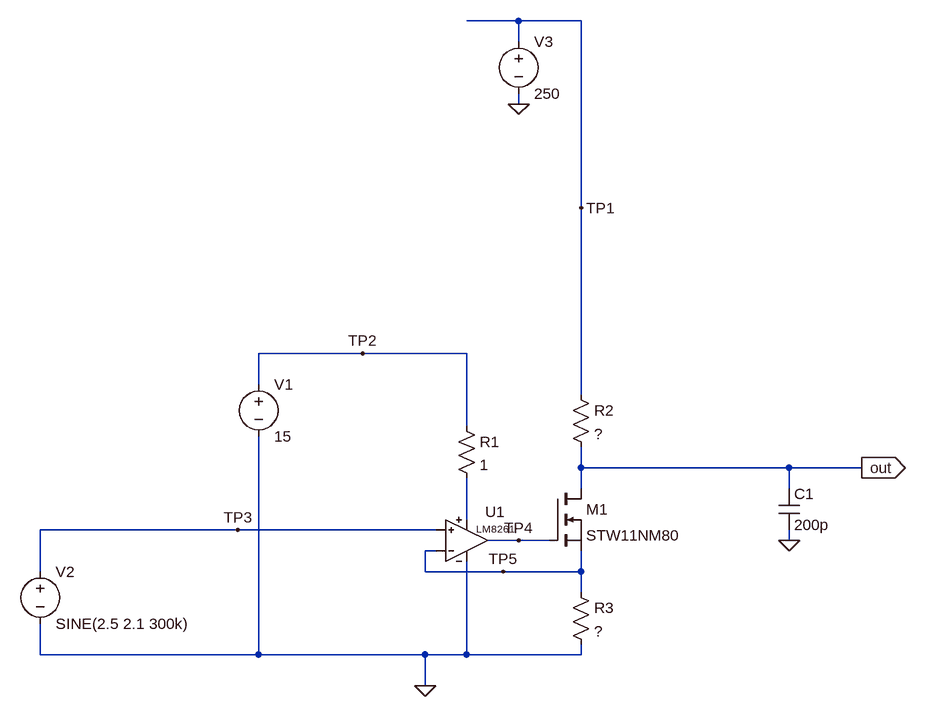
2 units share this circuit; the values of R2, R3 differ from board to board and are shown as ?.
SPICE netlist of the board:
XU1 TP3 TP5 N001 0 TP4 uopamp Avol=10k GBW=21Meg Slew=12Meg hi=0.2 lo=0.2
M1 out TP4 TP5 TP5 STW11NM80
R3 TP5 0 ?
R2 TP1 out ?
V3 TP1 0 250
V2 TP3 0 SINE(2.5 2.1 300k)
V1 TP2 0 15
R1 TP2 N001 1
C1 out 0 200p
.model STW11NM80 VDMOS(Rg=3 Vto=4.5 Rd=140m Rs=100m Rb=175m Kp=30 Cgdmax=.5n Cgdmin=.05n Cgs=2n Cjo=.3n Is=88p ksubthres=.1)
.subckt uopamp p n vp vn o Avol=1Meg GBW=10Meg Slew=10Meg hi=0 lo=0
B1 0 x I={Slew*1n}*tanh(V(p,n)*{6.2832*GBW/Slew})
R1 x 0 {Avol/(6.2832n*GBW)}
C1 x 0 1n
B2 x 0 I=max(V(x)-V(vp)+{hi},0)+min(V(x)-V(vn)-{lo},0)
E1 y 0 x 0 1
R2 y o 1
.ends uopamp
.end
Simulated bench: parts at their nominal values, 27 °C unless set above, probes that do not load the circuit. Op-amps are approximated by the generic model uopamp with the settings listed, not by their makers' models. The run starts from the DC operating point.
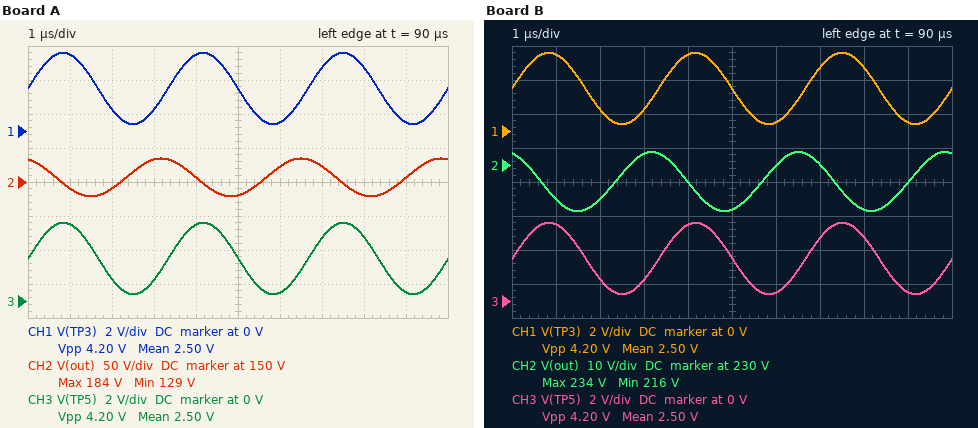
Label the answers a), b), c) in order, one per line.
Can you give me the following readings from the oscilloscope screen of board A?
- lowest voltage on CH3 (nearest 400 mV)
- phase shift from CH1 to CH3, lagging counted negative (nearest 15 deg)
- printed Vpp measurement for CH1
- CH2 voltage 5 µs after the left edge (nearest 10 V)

a) 400 mV
b) 0 deg
c) 4.20 V
d) 130 V
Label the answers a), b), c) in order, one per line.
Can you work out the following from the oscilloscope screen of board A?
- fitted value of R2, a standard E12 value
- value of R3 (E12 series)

a) 5.6 kΩ
b) 150 Ω
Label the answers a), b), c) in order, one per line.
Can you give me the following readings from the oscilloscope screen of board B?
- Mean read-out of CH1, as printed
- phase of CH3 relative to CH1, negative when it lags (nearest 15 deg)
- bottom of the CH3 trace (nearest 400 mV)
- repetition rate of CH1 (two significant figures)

a) 2.50 V
b) 0 deg
c) 400 mV
d) 300 kHz
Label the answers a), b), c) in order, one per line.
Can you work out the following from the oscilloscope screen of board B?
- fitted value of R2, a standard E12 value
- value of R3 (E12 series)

a) 4.7 kΩ
b) 470 Ω
